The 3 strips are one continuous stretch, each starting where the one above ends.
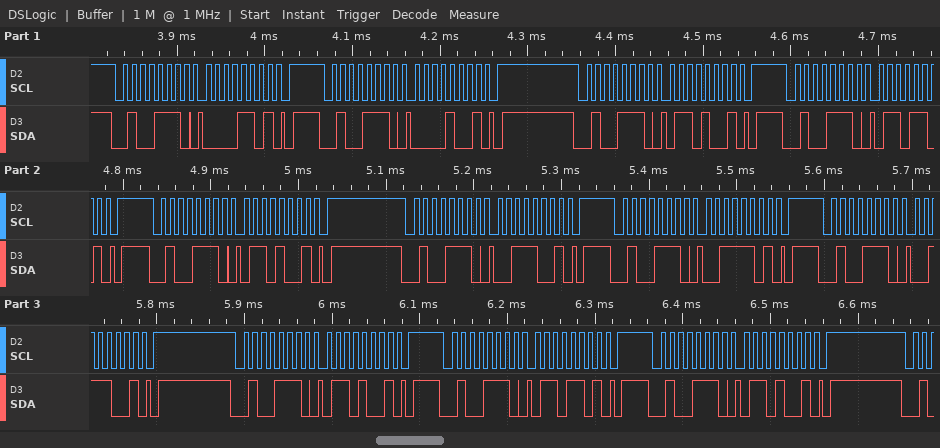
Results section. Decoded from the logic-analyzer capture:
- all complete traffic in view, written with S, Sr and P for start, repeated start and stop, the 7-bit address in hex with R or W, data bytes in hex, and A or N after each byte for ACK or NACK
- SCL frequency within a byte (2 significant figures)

S 27W A 0D A P S 27W A 09 A P S 27W A 69 A P S 27W A 6D A P S 27W A 69 A P S 27W A 39 A P S 27W A 3D A P S 27W A 39 A P S 27W A 69 A P S 27W A 6D A P S 27W A 69 A P
100 kHz
